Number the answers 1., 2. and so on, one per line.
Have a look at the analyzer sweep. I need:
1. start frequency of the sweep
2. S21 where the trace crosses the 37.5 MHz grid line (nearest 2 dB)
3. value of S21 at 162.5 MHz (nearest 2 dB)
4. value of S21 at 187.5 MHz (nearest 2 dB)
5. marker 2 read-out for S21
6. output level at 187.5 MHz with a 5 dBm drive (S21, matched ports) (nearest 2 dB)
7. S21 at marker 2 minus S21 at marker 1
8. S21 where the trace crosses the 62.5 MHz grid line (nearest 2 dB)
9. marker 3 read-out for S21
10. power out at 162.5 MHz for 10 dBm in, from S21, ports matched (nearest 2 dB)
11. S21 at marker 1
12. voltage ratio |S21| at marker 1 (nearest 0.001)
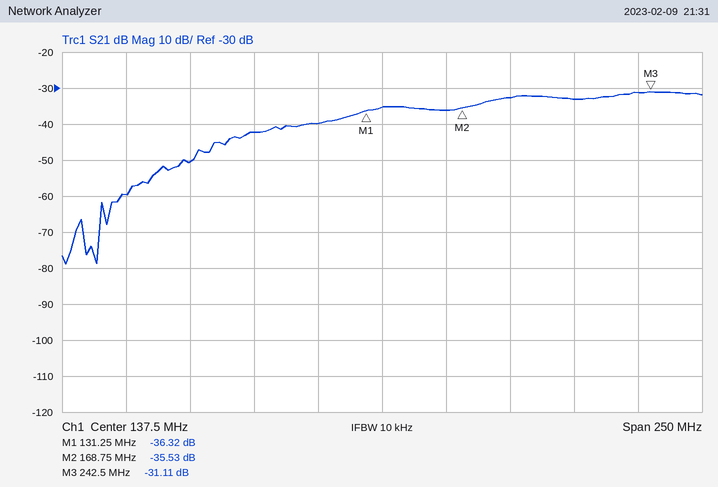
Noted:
1. 12.5 MHz
2. -60 dB
3. -36 dB
4. -32 dB
5. -35.53 dB
6. -28 dBm
7. 0.79 dB
8. -50 dB
9. -31.11 dB
10. -26 dBm
11. -36.32 dB
12. 0.015
